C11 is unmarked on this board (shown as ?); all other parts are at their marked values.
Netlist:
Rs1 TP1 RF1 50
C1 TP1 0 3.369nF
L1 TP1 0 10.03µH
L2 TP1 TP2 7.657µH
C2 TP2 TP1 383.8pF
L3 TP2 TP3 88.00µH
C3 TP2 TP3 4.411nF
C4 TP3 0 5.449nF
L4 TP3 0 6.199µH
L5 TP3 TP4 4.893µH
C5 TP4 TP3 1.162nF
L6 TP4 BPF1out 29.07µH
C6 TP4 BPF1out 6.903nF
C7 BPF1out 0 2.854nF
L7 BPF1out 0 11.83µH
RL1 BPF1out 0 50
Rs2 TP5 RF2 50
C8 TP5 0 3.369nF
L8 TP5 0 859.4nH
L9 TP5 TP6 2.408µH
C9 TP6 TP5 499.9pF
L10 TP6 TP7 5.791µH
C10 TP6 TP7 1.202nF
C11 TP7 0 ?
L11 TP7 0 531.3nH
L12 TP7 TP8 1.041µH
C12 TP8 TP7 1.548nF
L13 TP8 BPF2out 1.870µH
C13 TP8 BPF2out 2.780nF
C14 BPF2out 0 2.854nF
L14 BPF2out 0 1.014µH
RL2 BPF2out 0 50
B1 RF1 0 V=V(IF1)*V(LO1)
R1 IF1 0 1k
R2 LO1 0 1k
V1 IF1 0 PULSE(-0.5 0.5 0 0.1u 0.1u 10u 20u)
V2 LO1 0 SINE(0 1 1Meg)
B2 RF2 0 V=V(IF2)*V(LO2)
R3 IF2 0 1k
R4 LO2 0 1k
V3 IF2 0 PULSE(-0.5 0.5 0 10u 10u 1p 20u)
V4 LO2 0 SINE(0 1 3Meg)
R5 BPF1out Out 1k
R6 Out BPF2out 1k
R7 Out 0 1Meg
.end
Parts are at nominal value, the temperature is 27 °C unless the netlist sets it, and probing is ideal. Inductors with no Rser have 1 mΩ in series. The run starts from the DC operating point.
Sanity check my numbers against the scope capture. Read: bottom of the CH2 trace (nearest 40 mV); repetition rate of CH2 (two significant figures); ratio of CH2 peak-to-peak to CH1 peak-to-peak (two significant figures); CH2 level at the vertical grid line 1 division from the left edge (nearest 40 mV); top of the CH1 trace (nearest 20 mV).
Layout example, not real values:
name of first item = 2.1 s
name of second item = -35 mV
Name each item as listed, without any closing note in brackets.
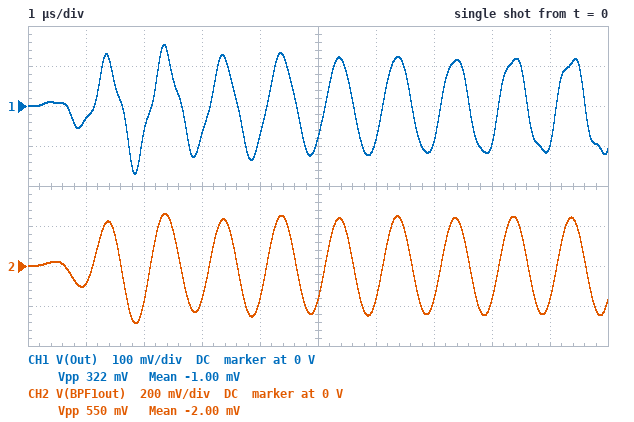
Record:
bottom of the CH2 trace = -280 mV
repetition rate of CH2 = 1.0 MHz
ratio of CH2 peak-to-peak to CH1 peak-to-peak = 1.7
CH2 level at the vertical grid line 1 division from the left edge = -80 mV
top of the CH1 trace = 160 mV
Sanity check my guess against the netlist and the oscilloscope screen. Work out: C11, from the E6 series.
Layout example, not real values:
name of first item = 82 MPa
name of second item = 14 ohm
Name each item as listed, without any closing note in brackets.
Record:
C11, from the E6 series = 15 nF
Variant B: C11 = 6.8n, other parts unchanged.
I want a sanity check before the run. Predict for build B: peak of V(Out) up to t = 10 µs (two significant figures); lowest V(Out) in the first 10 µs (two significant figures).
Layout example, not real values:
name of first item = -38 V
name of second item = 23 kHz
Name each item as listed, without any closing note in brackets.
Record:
peak of V(Out) up to t = 10 µs = 210 mV
lowest V(Out) in the first 10 µs = -240 mV
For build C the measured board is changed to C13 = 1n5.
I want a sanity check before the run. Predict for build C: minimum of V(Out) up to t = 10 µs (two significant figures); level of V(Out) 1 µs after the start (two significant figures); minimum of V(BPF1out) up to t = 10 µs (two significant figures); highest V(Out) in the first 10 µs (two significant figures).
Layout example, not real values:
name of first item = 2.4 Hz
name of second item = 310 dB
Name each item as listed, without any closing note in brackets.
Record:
minimum of V(Out) up to t = 10 µs = -140 mV
level of V(Out) 1 µs after the start = -40 mV
minimum of V(BPF1out) up to t = 10 µs = -290 mV
highest V(Out) in the first 10 µs = 130 mV
